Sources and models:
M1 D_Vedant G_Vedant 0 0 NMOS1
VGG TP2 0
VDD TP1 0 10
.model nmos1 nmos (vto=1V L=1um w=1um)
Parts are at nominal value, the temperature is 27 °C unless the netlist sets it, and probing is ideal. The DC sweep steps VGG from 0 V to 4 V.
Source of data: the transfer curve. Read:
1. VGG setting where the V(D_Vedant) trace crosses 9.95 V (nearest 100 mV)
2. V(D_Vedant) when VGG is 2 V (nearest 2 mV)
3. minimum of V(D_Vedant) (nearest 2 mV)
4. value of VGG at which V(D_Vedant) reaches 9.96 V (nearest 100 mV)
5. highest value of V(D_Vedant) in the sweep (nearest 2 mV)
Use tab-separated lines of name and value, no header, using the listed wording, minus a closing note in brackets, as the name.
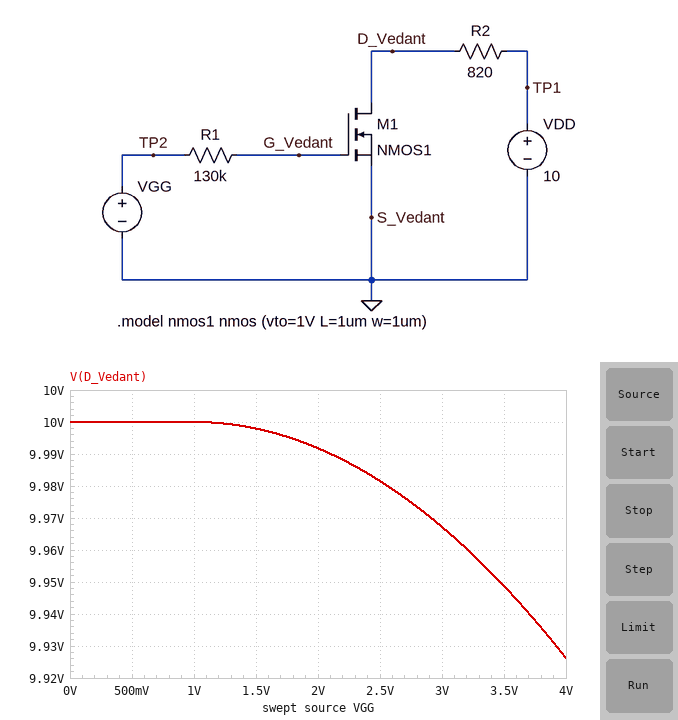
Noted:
VGG setting where the V(D_Vedant) trace crosses 9.95 V	3.5 V
V(D_Vedant) when VGG is 2 V	9.992 V
minimum of V(D_Vedant)	9.926 V
value of VGG at which V(D_Vedant) reaches 9.96 V	3.2 V
highest value of V(D_Vedant) in the sweep	10.000 V
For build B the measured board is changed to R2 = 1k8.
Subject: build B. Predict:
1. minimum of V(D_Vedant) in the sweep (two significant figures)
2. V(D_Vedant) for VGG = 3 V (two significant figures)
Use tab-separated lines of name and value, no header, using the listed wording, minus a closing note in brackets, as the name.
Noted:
minimum of V(D_Vedant) in the sweep	9.8 V
V(D_Vedant) for VGG = 3 V	9.9 V
